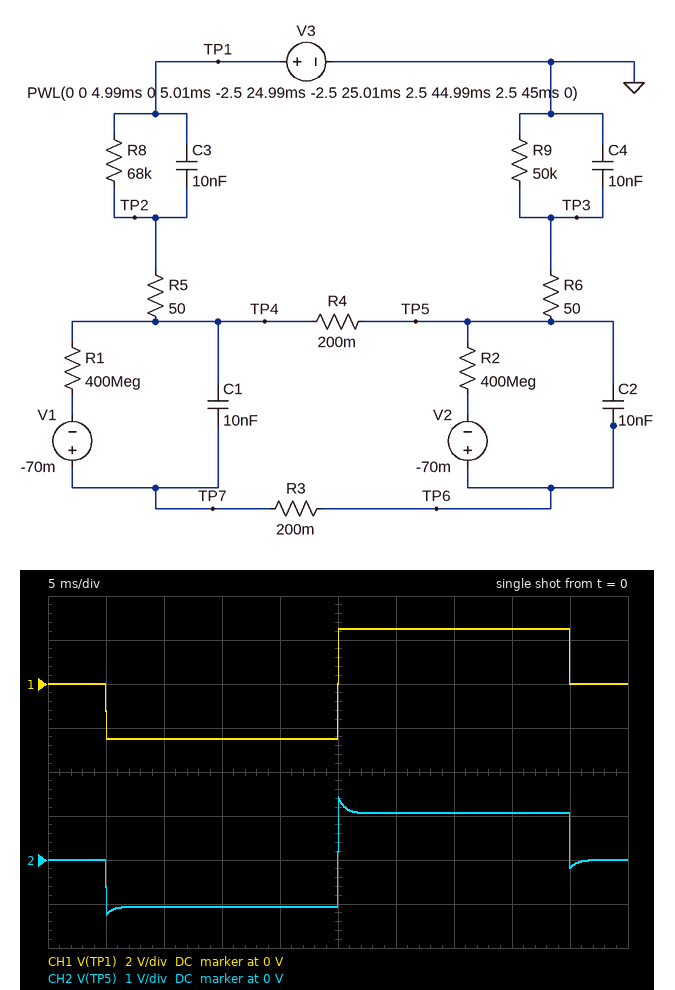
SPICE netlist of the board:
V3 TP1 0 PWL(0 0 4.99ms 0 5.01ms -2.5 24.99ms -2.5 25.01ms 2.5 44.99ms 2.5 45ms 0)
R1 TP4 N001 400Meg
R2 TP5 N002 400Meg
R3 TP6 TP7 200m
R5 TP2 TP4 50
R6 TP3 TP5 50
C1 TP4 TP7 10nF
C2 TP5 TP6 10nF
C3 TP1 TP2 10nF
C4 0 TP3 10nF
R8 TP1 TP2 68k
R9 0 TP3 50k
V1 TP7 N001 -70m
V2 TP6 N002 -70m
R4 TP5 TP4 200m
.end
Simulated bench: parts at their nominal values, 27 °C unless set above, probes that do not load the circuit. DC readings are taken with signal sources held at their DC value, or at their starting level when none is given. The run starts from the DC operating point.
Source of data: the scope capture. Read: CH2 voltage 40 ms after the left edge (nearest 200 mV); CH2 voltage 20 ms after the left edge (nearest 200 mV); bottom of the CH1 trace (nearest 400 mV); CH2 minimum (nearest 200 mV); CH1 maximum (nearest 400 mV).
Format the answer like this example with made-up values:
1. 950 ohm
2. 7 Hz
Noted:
1. 1.0 V
2. -1.0 V
3. -2.4 V
4. -1.2 V
5. 2.4 V
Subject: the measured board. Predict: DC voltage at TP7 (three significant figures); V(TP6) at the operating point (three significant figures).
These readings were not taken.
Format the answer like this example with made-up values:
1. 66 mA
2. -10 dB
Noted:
1. -70.0 mV
2. -70.0 mV
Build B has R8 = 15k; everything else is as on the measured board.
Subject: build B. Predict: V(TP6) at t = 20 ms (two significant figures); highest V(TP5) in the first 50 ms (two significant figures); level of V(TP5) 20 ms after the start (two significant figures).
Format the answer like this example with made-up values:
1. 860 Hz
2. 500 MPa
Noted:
1. -2.0 V
2. 1.9 V
3. -1.9 V
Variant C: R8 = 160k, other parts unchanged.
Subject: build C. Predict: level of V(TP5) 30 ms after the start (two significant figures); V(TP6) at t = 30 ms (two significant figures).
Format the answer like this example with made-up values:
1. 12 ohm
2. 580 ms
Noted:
1. 600 mV
2. 530 mV
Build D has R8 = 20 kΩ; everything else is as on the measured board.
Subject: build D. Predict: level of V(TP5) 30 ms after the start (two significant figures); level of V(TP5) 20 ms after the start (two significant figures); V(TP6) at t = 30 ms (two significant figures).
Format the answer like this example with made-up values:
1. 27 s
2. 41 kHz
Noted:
1. 1.8 V
2. -1.8 V
3. 1.7 V
